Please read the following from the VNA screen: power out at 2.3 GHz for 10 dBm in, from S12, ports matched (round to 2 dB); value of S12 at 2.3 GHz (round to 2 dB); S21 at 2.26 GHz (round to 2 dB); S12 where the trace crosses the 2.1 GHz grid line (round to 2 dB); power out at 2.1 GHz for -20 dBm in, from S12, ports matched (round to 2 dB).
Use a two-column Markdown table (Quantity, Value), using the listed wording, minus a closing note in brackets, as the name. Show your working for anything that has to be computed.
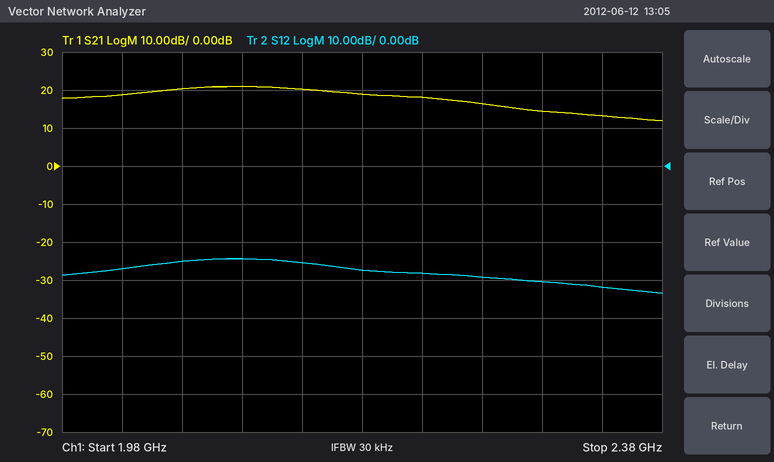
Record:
| Quantity | Value |
|---|---|
| power out at 2.3 GHz for 10 dBm in, from S12, ports matched | 10 dBm + (-30 dB) = -20 dBm |
| value of S12 at 2.3 GHz | -30 dB |
| S21 at 2.26 GHz | 16 dB |
| S12 where the trace crosses the 2.1 GHz grid line | -24 dB |
| power out at 2.1 GHz for -20 dBm in, from S12, ports matched | -20 dBm + (-24 dB) = -44 dBm |
